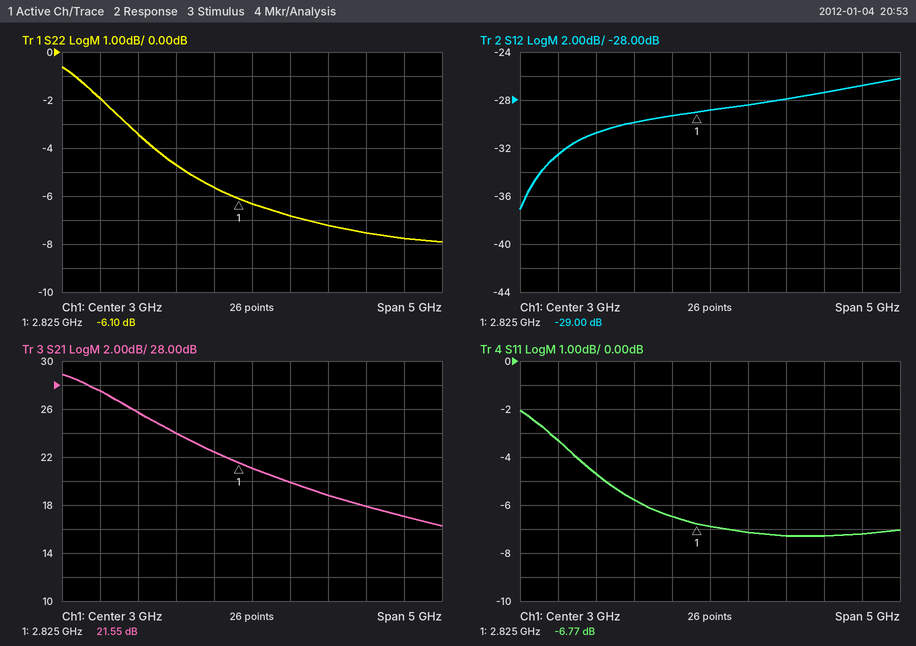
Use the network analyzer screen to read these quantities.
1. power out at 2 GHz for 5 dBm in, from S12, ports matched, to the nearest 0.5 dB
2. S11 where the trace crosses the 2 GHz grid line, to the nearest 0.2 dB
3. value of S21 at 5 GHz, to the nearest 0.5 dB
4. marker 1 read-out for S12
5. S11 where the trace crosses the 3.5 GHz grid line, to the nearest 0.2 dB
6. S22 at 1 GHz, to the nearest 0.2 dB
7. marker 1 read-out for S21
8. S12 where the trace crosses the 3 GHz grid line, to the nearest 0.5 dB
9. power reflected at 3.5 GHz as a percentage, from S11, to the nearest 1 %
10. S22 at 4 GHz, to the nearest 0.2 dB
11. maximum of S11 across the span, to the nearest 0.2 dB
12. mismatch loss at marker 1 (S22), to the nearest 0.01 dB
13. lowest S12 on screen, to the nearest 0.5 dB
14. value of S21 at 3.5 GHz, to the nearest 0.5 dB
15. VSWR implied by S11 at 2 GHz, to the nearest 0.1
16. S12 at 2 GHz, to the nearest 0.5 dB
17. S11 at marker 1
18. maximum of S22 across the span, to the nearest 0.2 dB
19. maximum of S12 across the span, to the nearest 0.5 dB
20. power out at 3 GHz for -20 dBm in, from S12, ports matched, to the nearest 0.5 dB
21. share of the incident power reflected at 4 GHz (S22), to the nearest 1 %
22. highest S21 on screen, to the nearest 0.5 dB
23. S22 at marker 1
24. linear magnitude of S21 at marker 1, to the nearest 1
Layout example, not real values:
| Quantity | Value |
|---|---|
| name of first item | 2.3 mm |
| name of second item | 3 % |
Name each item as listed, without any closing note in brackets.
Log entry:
| Quantity | Value |
|---|---|
| power out at 2 GHz for 5 dBm in, from S12, ports matched, to the nearest 0.5 dB | -25.0 dBm |
| S11 where the trace crosses the 2 GHz grid line, to the nearest 0.2 dB | -5.8 dB |
| value of S21 at 5 GHz, to the nearest 0.5 dB | 17.0 dB |
| marker 1 read-out for S12 | -29.00 dB |
| S11 where the trace crosses the 3.5 GHz grid line, to the nearest 0.2 dB | -7.2 dB |
| S22 at 1 GHz, to the nearest 0.2 dB | -2.0 dB |
| marker 1 read-out for S21 | 21.55 dB |
| S12 where the trace crosses the 3 GHz grid line, to the nearest 0.5 dB | -29.0 dB |
| power reflected at 3.5 GHz as a percentage, from S11, to the nearest 1 % | 19 % |
| S22 at 4 GHz, to the nearest 0.2 dB | -7.2 dB |
| maximum of S11 across the span, to the nearest 0.2 dB | -2.0 dB |
| mismatch loss at marker 1 (S22), to the nearest 0.01 dB | 1.22 dB |
| lowest S12 on screen, to the nearest 0.5 dB | -37.0 dB |
| value of S21 at 3.5 GHz, to the nearest 0.5 dB | 20.0 dB |
| VSWR implied by S11 at 2 GHz, to the nearest 0.1 | 3.1 |
| S12 at 2 GHz, to the nearest 0.5 dB | -30.0 dB |
| S11 at marker 1 | -6.77 dB |
| maximum of S22 across the span, to the nearest 0.2 dB | -0.6 dB |
| maximum of S12 across the span, to the nearest 0.5 dB | -26.0 dB |
| power out at 3 GHz for -20 dBm in, from S12, ports matched, to the nearest 0.5 dB | -49.0 dBm |
| share of the incident power reflected at 4 GHz (S22), to the nearest 1 % | 19 % |
| highest S21 on screen, to the nearest 0.5 dB | 29.0 dB |
| S22 at marker 1 | -6.10 dB |
| linear magnitude of S21 at marker 1, to the nearest 1 | 12 |
